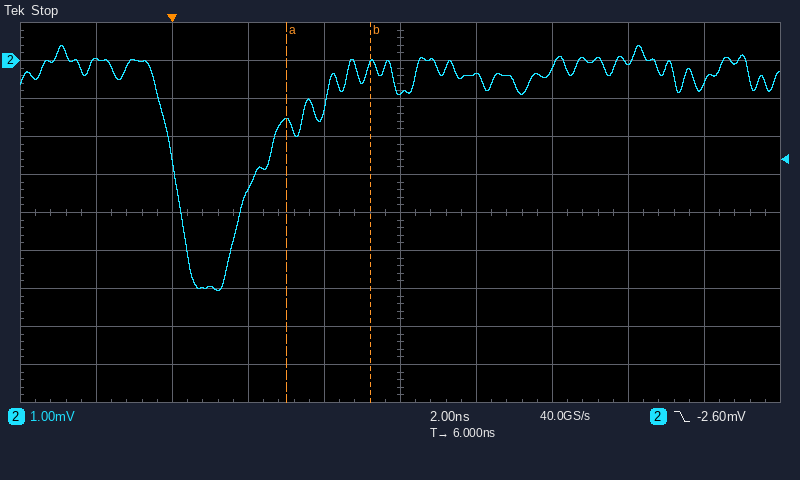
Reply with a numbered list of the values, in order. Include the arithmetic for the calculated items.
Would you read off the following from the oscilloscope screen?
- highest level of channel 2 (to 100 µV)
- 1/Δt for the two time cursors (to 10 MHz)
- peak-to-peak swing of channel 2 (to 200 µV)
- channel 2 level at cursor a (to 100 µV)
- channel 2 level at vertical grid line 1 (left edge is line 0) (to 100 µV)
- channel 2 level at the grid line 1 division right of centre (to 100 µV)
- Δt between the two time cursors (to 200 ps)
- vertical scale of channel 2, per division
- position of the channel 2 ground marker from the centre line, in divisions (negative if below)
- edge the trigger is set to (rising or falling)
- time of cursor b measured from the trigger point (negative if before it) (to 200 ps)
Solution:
1. 400 µV
2. 1 / 2.2 ns ≈ 450 MHz
3. 6.4 mV
4. -1.6 mV
5. 0.0 mV
6. -400 µV
7. 2.2 ns
8. 1 mV
9. +4.0 div
10. falling
11. +5.2 ns
